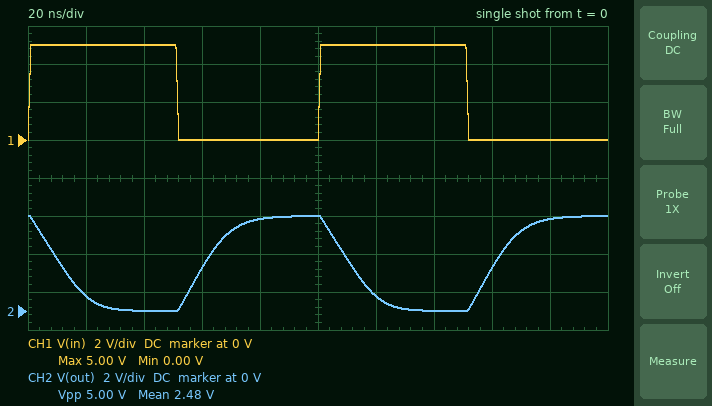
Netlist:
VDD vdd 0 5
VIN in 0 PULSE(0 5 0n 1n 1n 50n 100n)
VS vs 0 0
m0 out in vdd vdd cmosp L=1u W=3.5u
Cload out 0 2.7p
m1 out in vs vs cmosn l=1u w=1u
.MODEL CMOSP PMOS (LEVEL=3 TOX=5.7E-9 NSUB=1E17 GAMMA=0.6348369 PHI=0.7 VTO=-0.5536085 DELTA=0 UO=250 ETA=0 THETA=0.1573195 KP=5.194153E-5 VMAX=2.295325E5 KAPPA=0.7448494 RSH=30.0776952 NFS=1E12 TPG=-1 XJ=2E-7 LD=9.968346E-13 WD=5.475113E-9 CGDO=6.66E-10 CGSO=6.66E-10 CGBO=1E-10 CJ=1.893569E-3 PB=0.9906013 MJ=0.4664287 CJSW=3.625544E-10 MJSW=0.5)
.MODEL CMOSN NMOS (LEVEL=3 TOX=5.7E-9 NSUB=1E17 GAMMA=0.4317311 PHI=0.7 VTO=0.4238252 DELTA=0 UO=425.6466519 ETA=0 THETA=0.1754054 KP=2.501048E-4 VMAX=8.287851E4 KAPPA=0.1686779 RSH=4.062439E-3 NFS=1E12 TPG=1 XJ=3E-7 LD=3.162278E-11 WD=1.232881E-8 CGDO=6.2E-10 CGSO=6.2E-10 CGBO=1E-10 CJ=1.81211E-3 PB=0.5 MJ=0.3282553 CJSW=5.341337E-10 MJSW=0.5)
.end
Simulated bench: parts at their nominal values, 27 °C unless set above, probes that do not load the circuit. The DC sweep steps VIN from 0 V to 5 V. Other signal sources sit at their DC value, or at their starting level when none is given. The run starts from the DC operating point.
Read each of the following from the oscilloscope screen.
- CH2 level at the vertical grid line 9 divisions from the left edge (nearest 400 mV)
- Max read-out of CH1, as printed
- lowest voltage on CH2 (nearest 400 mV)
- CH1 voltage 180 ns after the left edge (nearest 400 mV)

4.8 V
5.00 V
0 V
0 V
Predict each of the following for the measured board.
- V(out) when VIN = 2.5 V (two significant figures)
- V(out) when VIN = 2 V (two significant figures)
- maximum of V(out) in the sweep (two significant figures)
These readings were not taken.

1.1 V
4.4 V
5.0 V
